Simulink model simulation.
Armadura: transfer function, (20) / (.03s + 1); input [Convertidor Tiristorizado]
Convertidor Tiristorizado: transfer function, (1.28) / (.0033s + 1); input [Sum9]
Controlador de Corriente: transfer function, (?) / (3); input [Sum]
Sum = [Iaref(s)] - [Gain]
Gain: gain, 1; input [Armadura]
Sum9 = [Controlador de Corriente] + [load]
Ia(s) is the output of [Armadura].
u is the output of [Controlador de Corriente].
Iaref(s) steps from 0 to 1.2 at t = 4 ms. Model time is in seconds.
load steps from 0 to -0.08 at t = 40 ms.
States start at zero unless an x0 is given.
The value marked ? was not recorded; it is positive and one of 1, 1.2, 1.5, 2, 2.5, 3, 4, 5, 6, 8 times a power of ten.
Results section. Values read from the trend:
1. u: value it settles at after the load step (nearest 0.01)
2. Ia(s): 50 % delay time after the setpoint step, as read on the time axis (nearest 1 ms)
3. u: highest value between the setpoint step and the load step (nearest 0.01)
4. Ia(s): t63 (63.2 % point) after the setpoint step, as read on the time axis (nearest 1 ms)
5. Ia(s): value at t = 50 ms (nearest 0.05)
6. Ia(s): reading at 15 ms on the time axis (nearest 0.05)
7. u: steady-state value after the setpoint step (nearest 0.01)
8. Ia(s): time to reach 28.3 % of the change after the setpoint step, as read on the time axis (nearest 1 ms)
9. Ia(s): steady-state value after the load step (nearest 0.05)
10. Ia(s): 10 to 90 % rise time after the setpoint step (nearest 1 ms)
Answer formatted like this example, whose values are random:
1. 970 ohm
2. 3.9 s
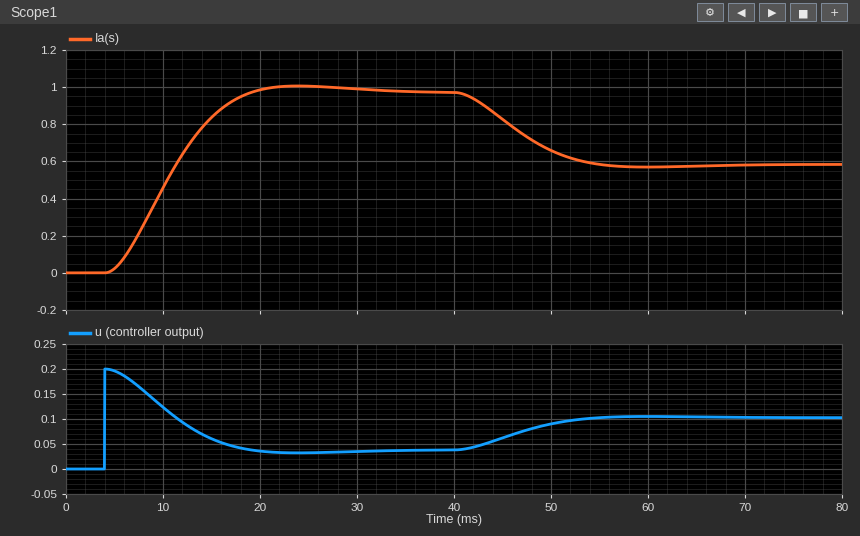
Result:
1. 0.10
2. 10 ms
3. 0.20
4. 12 ms
5. 0.65
6. 0.85
7. 0.04
8. 8 ms
9. 0.60
10. 10 ms
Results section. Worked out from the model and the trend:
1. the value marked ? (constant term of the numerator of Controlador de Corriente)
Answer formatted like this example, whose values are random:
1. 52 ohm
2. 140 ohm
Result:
1. 0.5
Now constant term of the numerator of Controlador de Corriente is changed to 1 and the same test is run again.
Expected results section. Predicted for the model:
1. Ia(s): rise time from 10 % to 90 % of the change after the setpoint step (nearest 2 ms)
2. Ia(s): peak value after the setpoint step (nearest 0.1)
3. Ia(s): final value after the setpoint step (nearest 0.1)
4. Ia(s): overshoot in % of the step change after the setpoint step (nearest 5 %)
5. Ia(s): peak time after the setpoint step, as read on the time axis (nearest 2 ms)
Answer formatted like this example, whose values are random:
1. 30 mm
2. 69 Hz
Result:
1. 6 ms
2. 1.2
3. 1.1
4. 15 %
5. 16 ms
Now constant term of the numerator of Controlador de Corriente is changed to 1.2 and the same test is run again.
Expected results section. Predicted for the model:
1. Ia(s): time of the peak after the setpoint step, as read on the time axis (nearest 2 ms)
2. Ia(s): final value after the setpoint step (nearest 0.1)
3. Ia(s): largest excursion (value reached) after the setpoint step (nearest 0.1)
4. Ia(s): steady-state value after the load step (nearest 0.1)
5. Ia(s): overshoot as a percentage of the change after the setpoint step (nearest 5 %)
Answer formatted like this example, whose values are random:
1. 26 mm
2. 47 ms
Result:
1. 14 ms
2. 1.1
3. 1.3
4. 0.9
5. 15 %
